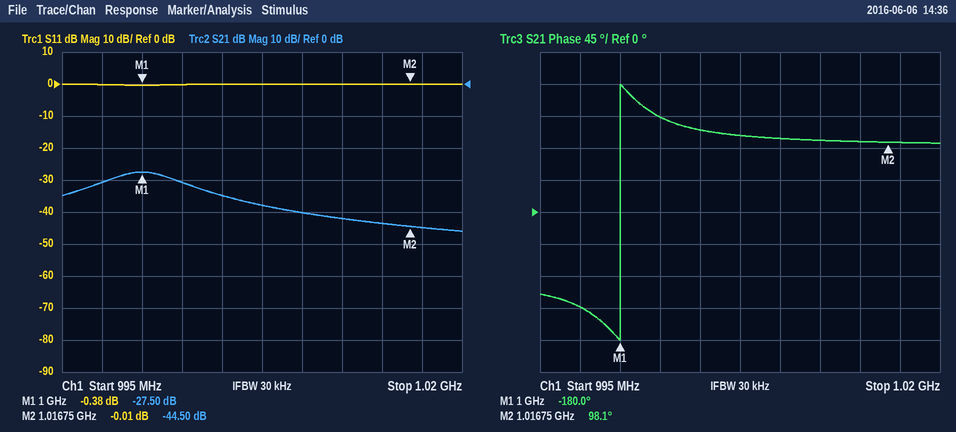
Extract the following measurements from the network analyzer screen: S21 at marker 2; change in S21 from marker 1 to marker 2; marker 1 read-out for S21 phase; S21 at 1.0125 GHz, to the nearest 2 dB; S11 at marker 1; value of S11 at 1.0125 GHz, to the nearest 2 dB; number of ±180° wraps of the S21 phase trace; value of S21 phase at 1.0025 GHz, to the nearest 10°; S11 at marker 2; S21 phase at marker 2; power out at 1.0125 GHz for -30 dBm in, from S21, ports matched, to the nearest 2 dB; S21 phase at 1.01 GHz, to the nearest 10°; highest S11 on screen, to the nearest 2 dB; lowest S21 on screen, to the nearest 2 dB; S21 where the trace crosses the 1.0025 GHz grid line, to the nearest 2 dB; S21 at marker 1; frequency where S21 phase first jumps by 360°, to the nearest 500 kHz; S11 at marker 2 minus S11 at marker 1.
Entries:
-44.50 dB
-17.00 dB
-180.0°
-42 dB
-0.38 dB
0 dB
1
130°
-0.01 dB
98.1°
-72 dBm
100°
0 dB
-46 dB
-30 dB
-27.50 dB
1.0000 GHz
0.37 dB
